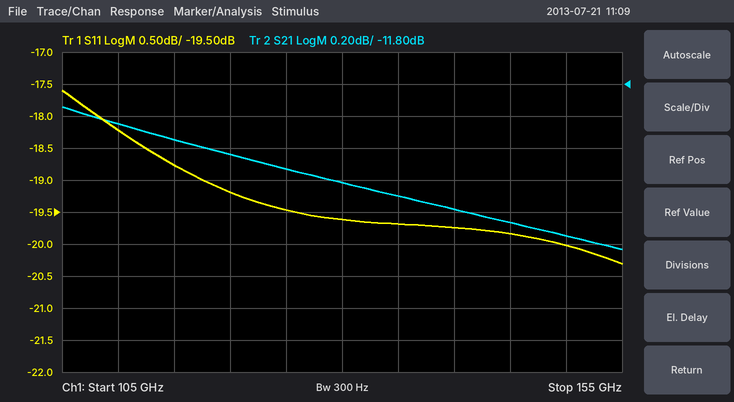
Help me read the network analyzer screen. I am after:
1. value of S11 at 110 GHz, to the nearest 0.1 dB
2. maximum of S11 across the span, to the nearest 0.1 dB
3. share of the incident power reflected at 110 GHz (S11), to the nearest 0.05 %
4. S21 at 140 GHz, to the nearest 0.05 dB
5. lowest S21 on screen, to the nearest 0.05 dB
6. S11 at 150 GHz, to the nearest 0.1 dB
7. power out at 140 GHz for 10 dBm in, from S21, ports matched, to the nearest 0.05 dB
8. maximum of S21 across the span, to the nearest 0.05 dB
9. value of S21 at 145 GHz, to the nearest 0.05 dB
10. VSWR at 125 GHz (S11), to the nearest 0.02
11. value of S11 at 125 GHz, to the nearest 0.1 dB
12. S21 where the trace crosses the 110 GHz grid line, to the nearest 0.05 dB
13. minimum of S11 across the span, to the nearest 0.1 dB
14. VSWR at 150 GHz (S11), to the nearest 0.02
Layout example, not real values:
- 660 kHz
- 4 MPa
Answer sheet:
- -18.2 dB
- -17.6 dB
- 1.50 %
- -12.60 dB
- -12.85 dB
- -20.0 dB
- -2.60 dBm
- -11.95 dB
- -12.65 dB
- 1.24
- -19.5 dB
- -12.05 dB
- -20.3 dB
- 1.22
